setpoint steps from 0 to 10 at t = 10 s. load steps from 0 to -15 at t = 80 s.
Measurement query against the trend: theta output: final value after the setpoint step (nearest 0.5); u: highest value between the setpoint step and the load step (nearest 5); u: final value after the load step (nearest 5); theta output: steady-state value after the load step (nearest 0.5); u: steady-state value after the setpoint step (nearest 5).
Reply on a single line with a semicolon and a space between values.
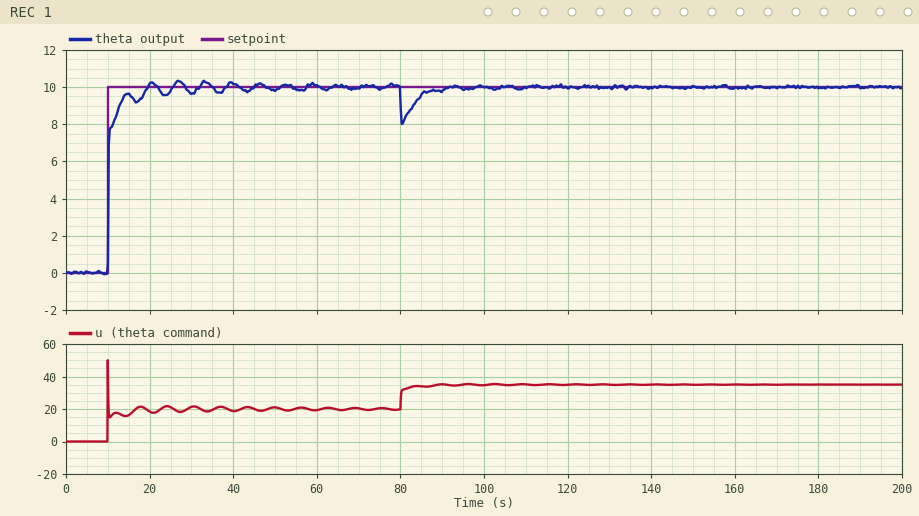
10.0; 50; 35; 10.0; 20
